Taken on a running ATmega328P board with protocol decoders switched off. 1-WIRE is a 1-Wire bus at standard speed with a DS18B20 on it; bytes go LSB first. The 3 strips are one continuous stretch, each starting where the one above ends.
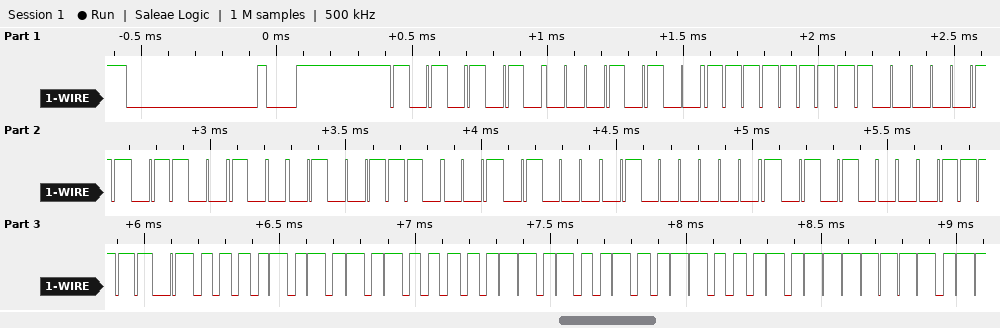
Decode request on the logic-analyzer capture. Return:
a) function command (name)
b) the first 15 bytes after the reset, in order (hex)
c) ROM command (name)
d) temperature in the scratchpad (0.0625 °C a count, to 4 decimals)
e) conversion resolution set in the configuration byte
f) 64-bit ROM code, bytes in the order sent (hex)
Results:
Read Scratchpad
55 28 FF C1 26 72 14 02 15 BE 50 05 4B 46 7F
Match ROM
85.0000 °C
12 bits
28 FF C1 26 72 14 02 15
